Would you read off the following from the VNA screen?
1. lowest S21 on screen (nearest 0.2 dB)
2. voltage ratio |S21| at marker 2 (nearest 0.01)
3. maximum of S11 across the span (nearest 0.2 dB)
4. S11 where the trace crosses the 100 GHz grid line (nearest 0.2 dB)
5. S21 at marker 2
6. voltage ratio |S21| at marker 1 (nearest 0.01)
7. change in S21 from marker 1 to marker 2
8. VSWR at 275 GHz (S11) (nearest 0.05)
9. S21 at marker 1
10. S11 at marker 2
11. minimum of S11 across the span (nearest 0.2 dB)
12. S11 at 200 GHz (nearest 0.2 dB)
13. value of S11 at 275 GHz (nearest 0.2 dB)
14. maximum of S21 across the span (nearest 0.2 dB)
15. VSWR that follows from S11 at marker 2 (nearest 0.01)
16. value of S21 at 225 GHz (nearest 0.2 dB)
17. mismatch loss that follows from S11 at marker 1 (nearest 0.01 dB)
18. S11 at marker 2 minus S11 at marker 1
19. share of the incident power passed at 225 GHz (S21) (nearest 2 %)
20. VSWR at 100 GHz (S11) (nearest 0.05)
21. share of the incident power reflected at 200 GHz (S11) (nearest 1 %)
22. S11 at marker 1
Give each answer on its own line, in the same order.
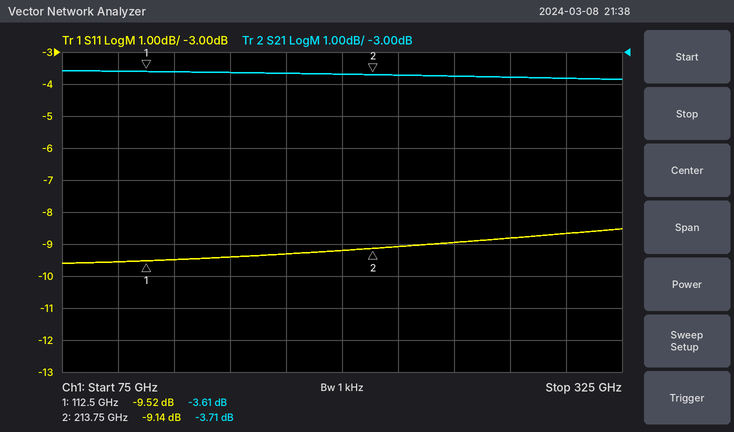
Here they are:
-3.8 dB
0.65
-8.6 dB
-9.6 dB
-3.71 dB
0.66
-0.10 dB
2.15
-3.61 dB
-9.14 dB
-9.6 dB
-9.2 dB
-8.8 dB
-3.6 dB
2.07
-3.8 dB
0.51 dB
0.38 dB
42 %
2.00
12 %
-9.52 dB
